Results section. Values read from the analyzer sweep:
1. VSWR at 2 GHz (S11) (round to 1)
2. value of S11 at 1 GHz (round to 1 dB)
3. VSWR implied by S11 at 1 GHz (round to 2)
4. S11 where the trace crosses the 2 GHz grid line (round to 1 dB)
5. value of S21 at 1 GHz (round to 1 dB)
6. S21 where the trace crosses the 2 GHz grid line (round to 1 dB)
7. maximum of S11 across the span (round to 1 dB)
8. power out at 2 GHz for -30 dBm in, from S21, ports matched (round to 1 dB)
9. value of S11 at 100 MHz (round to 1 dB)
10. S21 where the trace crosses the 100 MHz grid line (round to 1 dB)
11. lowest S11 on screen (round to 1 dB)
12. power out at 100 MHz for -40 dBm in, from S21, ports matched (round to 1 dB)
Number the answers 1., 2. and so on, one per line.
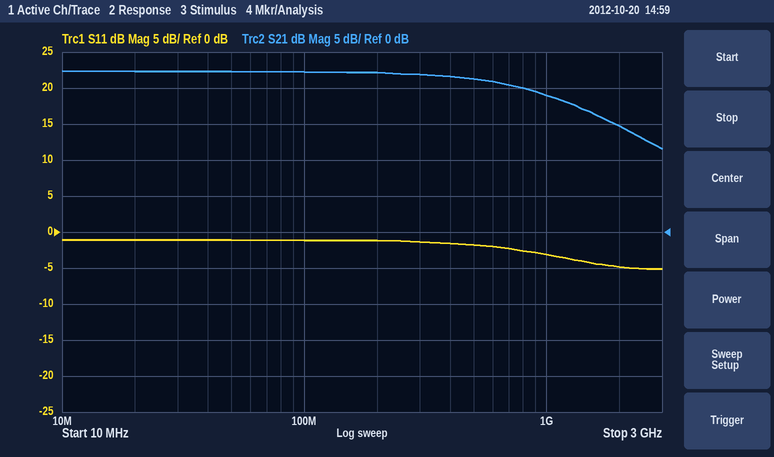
1. 4
2. -3 dB
3. 6
4. -5 dB
5. 19 dB
6. 15 dB
7. -1 dB
8. -15 dBm
9. -1 dB
10. 22 dB
11. -5 dB
12. -18 dBm
